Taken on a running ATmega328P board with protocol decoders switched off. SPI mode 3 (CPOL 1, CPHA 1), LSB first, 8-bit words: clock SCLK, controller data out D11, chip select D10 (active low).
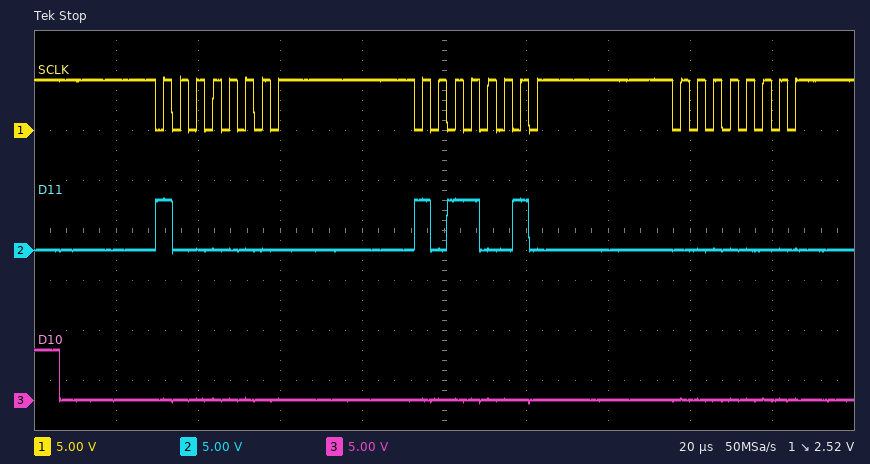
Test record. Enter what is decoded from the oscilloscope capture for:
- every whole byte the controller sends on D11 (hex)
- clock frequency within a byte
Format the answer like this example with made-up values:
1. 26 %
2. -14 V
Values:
1. 01 4D 00
2. 250 kHz
